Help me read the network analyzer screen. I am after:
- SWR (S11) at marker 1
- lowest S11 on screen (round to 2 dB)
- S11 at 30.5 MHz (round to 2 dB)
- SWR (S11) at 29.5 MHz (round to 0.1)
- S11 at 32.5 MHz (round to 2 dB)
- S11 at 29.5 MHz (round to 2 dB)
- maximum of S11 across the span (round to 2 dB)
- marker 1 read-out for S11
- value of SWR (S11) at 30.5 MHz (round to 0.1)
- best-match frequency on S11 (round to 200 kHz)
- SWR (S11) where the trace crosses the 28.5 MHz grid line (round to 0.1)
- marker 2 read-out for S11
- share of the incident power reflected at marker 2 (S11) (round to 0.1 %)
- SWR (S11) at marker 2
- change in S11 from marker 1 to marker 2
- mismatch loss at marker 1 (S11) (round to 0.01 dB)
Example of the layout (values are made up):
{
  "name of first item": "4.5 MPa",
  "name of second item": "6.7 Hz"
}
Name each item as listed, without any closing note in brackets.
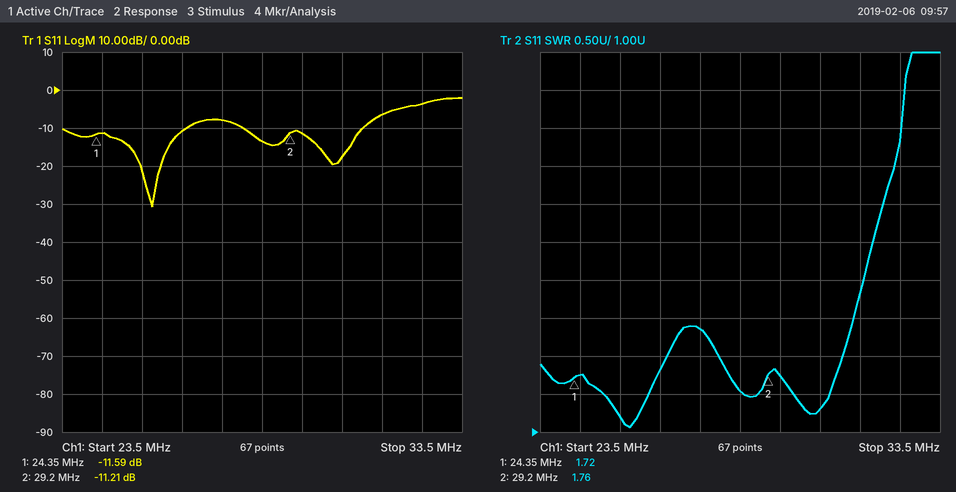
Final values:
{
  "SWR (S11) at marker 1": "1.72",
  "lowest S11 on screen": "-30 dB",
  "S11 at 30.5 MHz": "-18 dB",
  "SWR (S11) at 29.5 MHz": "1.7",
  "S11 at 32.5 MHz": "-4 dB",
  "S11 at 29.5 MHz": "-12 dB",
  "maximum of S11 across the span": "-2 dB",
  "marker 1 read-out for S11": "-11.59 dB",
  "value of SWR (S11) at 30.5 MHz": "1.3",
  "best-match frequency on S11": "25.8 MHz",
  "SWR (S11) where the trace crosses the 28.5 MHz grid line": "1.5",
  "marker 2 read-out for S11": "-11.21 dB",
  "share of the incident power reflected at marker 2 (S11)": "7.6 %",
  "SWR (S11) at marker 2": "1.76",
  "change in S11 from marker 1 to marker 2": "0.38 dB",
  "mismatch loss at marker 1 (S11)": "0.31 dB"
}
